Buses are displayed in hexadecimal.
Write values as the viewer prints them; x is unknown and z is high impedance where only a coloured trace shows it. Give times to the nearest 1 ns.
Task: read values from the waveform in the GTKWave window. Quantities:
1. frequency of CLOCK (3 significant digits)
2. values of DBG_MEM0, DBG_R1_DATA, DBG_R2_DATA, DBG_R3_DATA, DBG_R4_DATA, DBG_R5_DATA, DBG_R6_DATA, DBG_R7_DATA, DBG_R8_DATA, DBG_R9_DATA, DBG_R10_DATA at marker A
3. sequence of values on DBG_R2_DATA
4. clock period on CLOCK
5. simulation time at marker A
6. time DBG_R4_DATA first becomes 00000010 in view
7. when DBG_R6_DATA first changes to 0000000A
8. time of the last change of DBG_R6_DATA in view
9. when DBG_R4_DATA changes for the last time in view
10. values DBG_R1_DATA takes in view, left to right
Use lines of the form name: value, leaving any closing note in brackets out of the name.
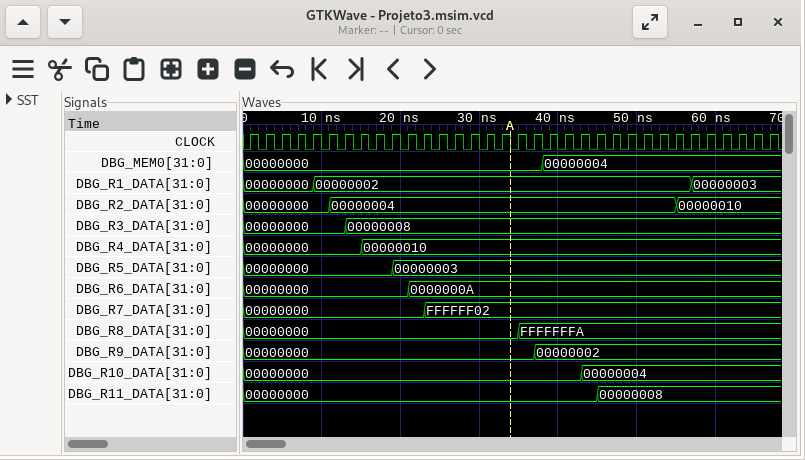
frequency of CLOCK: 500 MHz
values of DBG_MEM0, DBG_R1_DATA, DBG_R2_DATA, DBG_R3_DATA, DBG_R4_DATA, DBG_R5_DATA, DBG_R6_DATA, DBG_R7_DATA, DBG_R8_DATA, DBG_R9_DATA, DBG_R10_DATA at marker A: DBG_MEM0=00000000, DBG_R1_DATA=00000002, DBG_R2_DATA=00000004, DBG_R3_DATA=00000008, DBG_R4_DATA=00000010, DBG_R5_DATA=00000003, DBG_R6_DATA=0000000A, DBG_R7_DATA=FFFFFF02, DBG_R8_DATA=00000000, DBG_R9_DATA=00000000, DBG_R10_DATA=00000000
sequence of values on DBG_R2_DATA: 00000000, 00000004, 00000010
clock period on CLOCK: 2 ns
simulation time at marker A: 34 ns
time DBG_R4_DATA first becomes 00000010 in view: 15 ns
when DBG_R6_DATA first changes to 0000000A: 21 ns
time of the last change of DBG_R6_DATA in view: 21 ns
when DBG_R4_DATA changes for the last time in view: 15 ns
values DBG_R1_DATA takes in view, left to right: 00000000, 00000002, 00000003
